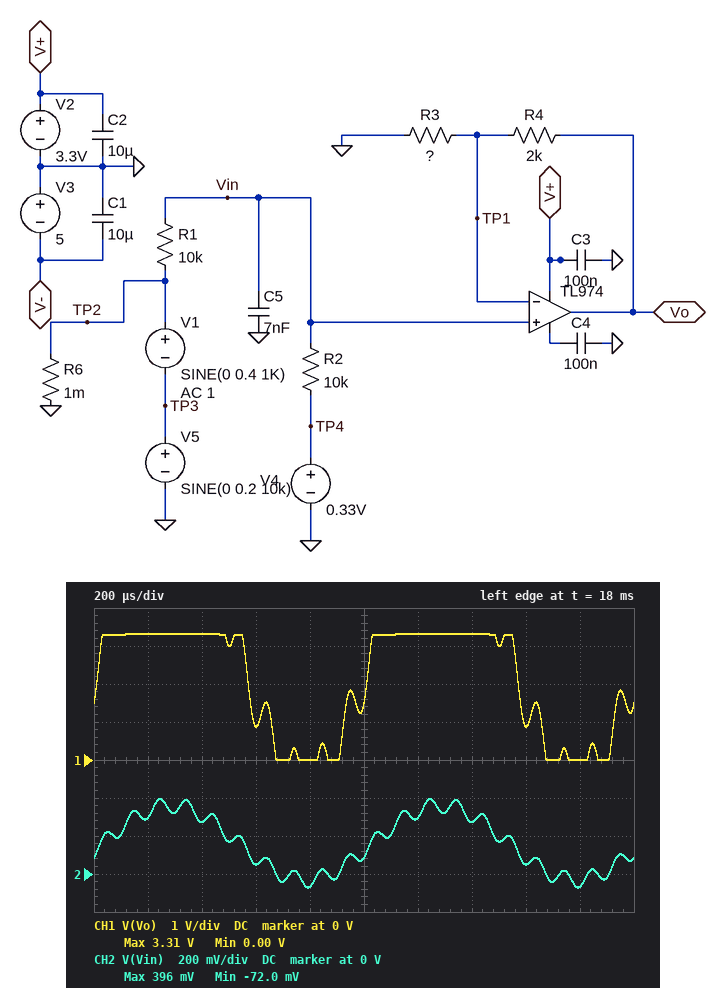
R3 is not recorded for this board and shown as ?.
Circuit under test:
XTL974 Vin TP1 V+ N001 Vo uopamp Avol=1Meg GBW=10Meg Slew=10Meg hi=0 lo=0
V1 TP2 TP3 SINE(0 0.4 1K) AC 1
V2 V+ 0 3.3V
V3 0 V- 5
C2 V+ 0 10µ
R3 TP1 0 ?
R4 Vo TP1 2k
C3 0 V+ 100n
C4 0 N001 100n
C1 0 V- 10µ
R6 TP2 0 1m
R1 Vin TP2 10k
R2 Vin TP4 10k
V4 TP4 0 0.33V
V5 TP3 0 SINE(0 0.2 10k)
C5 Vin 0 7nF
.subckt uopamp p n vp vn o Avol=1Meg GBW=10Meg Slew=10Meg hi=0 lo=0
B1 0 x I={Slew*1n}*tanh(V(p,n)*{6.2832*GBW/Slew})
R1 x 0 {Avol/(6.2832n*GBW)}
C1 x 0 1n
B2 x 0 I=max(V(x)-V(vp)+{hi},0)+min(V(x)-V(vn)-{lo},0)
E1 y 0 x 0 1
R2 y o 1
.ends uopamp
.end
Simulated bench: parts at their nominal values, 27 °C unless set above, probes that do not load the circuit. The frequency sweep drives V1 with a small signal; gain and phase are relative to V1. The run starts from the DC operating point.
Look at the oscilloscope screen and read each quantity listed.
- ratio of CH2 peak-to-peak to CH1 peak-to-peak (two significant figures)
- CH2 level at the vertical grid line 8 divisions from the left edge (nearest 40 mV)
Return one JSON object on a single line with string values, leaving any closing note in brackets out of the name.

{"ratio of CH2 peak-to-peak to CH1 peak-to-peak": "0.14", "CH2 level at the vertical grid line 8 divisions from the left edge": "40 mV"}
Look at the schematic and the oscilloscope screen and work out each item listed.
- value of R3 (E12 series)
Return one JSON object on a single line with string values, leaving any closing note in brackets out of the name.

{"value of R3": "120 Ω"}
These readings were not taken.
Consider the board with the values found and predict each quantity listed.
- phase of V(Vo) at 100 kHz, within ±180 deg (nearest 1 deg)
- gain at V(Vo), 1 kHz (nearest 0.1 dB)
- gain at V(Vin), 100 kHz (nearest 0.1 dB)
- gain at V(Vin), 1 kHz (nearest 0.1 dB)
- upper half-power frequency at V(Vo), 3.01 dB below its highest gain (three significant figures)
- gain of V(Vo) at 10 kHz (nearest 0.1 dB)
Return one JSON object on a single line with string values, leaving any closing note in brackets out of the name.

{"phase of V(Vo) at 100 kHz, within ±180 deg": "-97 deg", "gain at V(Vo), 1 kHz": "18.7 dB", "gain at V(Vin), 100 kHz": "-32.9 dB", "gain at V(Vin), 1 kHz": "-6.2 dB", "upper half-power frequency at V(Vo), 3.01 dB below its highest gain": "4.55 kHz", "gain of V(Vo) at 10 kHz": "11.3 dB"}
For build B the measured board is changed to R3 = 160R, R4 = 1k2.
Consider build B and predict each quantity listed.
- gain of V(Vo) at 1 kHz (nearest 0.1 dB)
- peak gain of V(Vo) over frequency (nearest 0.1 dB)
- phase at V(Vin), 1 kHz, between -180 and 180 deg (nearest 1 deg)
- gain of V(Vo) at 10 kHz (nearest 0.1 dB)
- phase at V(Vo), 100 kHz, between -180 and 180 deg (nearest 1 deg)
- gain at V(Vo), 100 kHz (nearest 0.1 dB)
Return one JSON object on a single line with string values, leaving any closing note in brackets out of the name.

{"gain of V(Vo) at 1 kHz": "12.4 dB", "peak gain of V(Vo) over frequency": "12.6 dB", "phase at V(Vin), 1 kHz, between -180 and 180 deg": "-12 deg", "gain of V(Vo) at 10 kHz": "4.9 dB", "phase at V(Vo), 100 kHz, between -180 and 180 deg": "-92 deg", "gain at V(Vo), 100 kHz": "-14.3 dB"}
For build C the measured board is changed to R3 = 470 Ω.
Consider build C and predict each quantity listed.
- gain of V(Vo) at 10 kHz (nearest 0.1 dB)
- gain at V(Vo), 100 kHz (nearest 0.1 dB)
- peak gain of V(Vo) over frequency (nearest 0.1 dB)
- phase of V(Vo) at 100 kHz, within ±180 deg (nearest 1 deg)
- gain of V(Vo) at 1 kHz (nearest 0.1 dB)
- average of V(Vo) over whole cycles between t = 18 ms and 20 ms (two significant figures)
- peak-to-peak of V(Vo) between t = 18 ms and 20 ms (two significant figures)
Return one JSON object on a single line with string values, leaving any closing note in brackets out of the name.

{"gain of V(Vo) at 10 kHz": "0.7 dB", "gain at V(Vo), 100 kHz": "-18.5 dB", "peak gain of V(Vo) over frequency": "8.4 dB", "phase of V(Vo) at 100 kHz, within ±180 deg": "-90 deg", "gain of V(Vo) at 1 kHz": "8.2 dB", "average of V(Vo) over whole cycles between t = 18 ms and 20 ms": "890 mV", "peak-to-peak of V(Vo) between t = 18 ms and 20 ms": "2.1 V"}
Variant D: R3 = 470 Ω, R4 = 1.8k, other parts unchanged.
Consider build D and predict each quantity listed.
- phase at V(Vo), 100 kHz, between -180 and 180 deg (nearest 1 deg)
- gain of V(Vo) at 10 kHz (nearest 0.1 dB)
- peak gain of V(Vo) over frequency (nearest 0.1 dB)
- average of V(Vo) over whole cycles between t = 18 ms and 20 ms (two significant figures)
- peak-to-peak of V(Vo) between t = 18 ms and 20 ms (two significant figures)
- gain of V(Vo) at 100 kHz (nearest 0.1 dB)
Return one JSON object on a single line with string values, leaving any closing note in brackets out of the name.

{"phase at V(Vo), 100 kHz, between -180 and 180 deg": "-90 deg", "gain of V(Vo) at 10 kHz": "0 dB", "peak gain of V(Vo) over frequency": "7.7 dB", "average of V(Vo) over whole cycles between t = 18 ms and 20 ms": "820 mV", "peak-to-peak of V(Vo) between t = 18 ms and 20 ms": "1.9 V", "gain of V(Vo) at 100 kHz": "-19.2 dB"}
